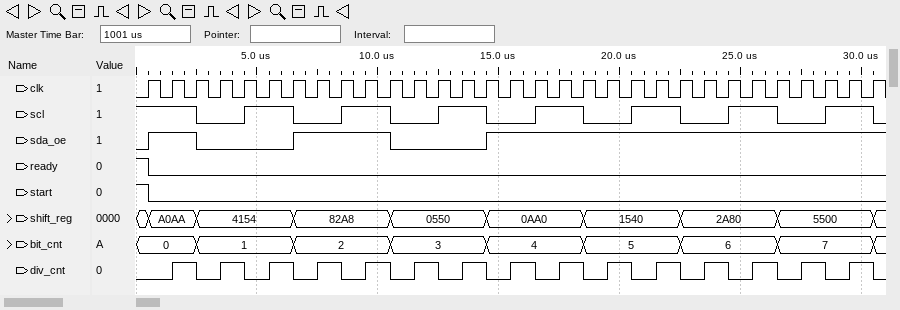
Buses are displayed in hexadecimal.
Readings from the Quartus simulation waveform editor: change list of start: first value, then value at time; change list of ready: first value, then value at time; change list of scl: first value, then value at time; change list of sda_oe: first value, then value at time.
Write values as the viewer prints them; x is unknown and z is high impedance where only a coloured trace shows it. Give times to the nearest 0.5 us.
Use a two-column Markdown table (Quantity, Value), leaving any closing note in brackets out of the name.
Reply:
| Quantity | Value |
|---|---|
| change list of start: first value, then value at time | 1, 0 at 0.5 us |
| change list of ready: first value, then value at time | 1, 0 at 0.5 us |
| change list of scl: first value, then value at time | 1, 0 at 2.5 us, 1 at 4.5 us, 0 at 6.5 us, 1 at 8.5 us, 0 at 10.5 us, 1 at 12.5 us, 0 at 14.5 us, 1 at 16.5 us, 0 at 18.5 us, 1 at 20.5 us, 0 at 22.5 us, 1 at 24.5 us, 0 at 26.5 us, 1 at 28.5 us, 0 at 30.5 us |
| change list of sda_oe: first value, then value at time | 0, 1 at 0.5 us, 0 at 2.5 us, 1 at 6.5 us, 0 at 10.5 us, 1 at 14.5 us |
